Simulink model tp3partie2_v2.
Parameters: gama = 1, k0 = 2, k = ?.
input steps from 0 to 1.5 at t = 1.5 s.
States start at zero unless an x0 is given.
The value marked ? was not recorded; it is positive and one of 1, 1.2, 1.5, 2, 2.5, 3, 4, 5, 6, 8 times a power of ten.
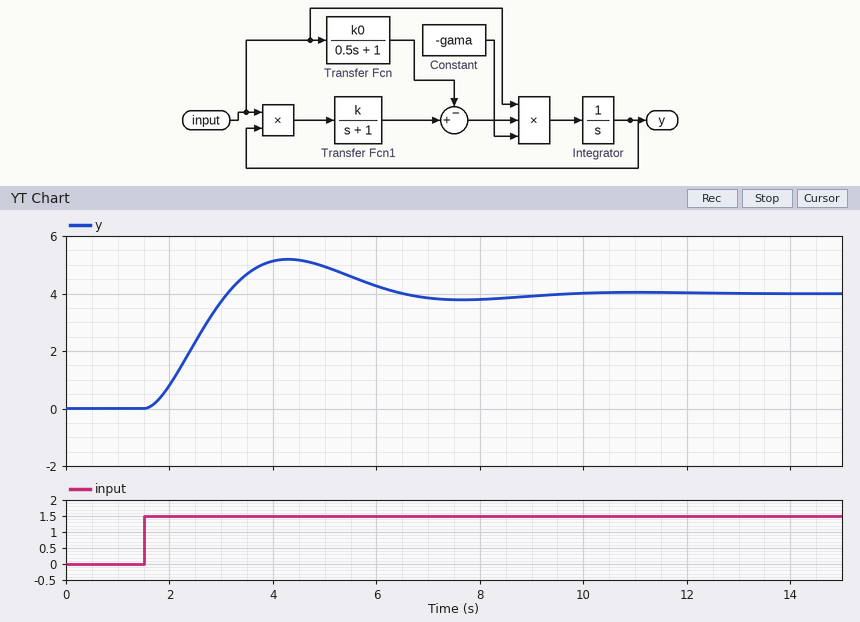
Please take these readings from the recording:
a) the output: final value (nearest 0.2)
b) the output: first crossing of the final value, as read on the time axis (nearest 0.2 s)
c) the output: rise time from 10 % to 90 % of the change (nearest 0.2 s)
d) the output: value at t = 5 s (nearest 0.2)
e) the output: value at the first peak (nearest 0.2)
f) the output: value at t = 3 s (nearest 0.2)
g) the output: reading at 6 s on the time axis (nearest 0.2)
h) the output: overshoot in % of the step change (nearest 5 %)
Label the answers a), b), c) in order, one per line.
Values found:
a) 4.0
b) 3.2 s
c) 1.2 s
d) 5.0
e) 5.2
f) 3.8
g) 4.2
h) 30 %
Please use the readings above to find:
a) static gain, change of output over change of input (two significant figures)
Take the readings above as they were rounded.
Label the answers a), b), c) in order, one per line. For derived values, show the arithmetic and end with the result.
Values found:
a) (4 - 0) / (1.5 - 0) = 2.7
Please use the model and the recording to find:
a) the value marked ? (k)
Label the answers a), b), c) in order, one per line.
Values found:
a) 0.5
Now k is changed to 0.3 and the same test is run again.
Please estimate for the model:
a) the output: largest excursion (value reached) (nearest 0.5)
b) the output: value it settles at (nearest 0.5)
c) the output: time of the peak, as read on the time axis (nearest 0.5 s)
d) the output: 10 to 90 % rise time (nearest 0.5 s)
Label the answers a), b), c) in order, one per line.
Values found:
a) 7.5
b) 6.5
c) 5.5 s
d) 2.0 s
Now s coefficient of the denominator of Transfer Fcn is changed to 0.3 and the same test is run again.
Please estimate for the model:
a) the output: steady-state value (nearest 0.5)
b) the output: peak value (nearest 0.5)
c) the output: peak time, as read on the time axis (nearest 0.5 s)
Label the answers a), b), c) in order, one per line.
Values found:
a) 4.0
b) 5.5
c) 4.0 s
